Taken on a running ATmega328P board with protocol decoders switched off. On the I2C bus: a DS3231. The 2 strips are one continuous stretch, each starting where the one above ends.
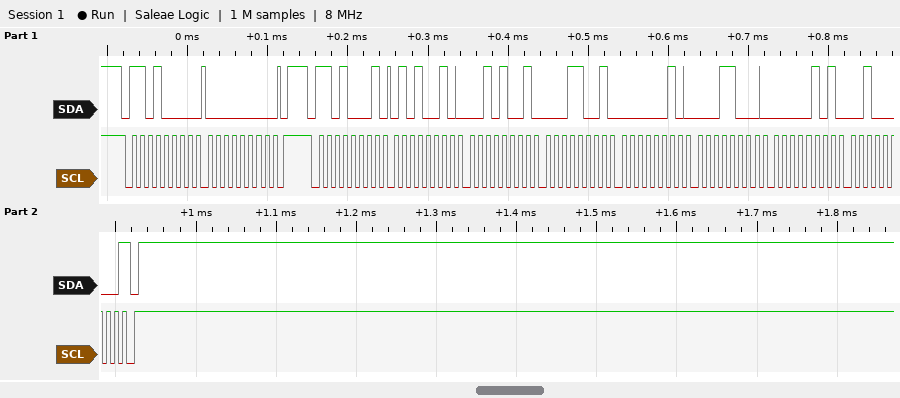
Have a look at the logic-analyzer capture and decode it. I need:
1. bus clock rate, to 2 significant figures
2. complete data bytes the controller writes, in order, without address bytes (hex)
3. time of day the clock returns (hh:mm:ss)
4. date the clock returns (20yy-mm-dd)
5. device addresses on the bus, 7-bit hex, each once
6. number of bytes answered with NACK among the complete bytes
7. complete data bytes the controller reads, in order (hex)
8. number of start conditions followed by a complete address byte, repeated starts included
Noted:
100 kHz
00
19:29:52
2020-05-18
0x68
1
52 29 19 02 18 05 20
2
